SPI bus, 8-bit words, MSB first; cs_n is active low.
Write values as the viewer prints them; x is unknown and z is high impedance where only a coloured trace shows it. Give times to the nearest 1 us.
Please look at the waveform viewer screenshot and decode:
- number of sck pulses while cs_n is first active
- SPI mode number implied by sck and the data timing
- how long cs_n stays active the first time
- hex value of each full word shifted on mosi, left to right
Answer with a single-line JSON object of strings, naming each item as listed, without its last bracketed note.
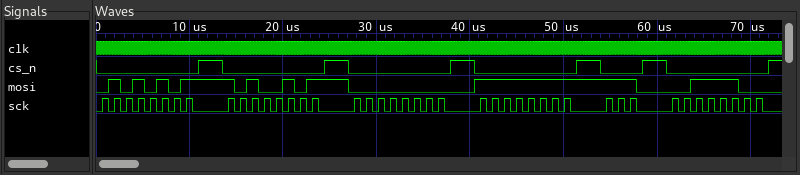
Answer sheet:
{"number of sck pulses while cs_n is first active": "8", "SPI mode number implied by sck and the data timing": "0", "how long cs_n stays active the first time": "11 us", "hex value of each full word shifted on mosi, left to right": "55, A5, 00, FF, 3C"}
